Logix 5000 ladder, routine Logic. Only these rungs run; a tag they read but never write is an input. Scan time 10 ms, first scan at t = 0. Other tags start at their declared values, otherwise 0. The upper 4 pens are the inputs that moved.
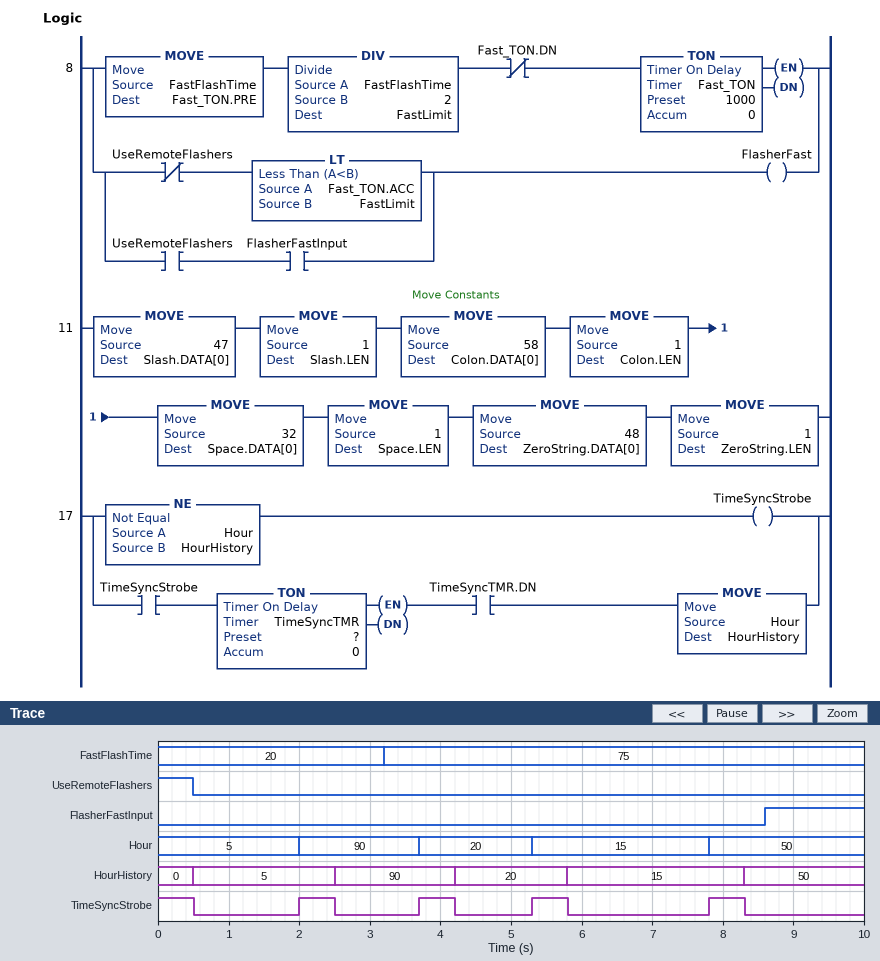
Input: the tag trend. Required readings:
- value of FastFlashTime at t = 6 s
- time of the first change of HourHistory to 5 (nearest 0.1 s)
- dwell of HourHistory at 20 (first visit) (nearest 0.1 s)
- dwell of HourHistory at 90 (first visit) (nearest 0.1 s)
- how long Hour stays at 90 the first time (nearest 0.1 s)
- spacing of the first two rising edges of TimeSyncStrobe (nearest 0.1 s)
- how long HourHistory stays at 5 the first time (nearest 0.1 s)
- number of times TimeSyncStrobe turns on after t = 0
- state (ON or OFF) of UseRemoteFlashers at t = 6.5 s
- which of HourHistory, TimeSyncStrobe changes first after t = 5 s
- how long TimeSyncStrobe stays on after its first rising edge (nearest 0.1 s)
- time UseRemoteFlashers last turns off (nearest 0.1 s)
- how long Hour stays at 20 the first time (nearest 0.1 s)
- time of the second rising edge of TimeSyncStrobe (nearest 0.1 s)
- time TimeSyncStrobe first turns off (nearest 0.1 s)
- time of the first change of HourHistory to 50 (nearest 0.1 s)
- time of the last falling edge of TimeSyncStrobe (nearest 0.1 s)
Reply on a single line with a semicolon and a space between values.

75; 0.5 s; 1.6 s; 1.7 s; 1.7 s; 1.7 s; 2.0 s; 4; OFF; TimeSyncStrobe; 0.5 s; 0.5 s; 1.6 s; 3.7 s; 0.5 s; 8.3 s; 8.3 s
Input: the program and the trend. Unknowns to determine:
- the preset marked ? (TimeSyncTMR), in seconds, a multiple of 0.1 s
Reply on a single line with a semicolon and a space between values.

0.5 s
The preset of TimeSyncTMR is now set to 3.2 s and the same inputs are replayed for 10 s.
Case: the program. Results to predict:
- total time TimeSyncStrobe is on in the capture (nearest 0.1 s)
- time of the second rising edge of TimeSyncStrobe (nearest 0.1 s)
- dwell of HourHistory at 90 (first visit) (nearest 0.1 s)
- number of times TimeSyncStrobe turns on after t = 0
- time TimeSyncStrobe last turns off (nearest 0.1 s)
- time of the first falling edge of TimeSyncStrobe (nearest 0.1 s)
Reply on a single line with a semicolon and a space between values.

8.6 s; 7.8 s; 3.7 s; 2; 6.9 s; 3.2 s
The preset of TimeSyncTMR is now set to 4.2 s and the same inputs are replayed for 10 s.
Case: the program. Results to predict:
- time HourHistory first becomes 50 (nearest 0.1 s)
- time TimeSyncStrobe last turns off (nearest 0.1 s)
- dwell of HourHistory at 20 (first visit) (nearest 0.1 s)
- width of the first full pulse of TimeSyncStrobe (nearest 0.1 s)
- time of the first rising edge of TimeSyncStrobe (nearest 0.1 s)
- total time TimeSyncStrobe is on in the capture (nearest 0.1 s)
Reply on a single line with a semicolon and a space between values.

9.5 s; 9.5 s; 5.3 s; 4.2 s; 5.3 s; 8.4 s
